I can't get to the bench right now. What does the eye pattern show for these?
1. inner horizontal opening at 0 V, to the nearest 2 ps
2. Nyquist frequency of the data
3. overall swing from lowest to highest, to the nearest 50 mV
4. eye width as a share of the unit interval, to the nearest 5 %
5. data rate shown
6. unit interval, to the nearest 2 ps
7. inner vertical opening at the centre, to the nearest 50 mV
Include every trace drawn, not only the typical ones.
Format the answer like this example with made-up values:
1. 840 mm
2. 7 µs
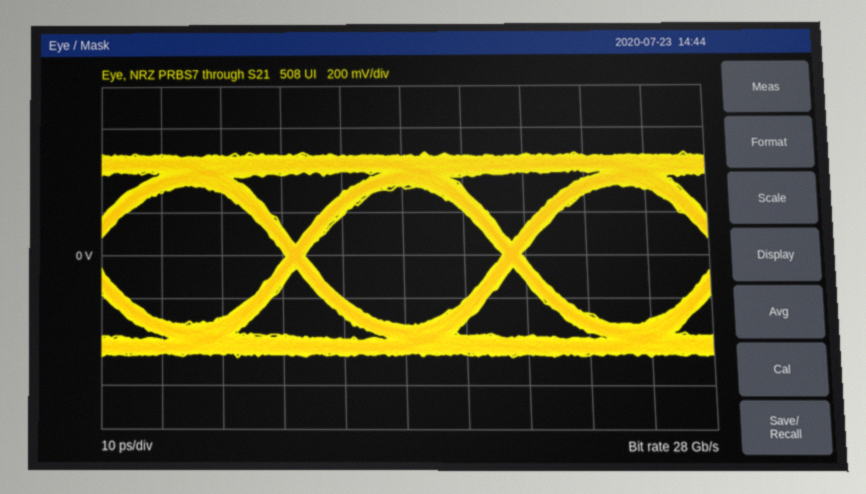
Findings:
1. 32 ps
2. 14 GHz
3. 950 mV
4. 90 %
5. 28 Gb/s
6. 36 ps
7. 650 mV
